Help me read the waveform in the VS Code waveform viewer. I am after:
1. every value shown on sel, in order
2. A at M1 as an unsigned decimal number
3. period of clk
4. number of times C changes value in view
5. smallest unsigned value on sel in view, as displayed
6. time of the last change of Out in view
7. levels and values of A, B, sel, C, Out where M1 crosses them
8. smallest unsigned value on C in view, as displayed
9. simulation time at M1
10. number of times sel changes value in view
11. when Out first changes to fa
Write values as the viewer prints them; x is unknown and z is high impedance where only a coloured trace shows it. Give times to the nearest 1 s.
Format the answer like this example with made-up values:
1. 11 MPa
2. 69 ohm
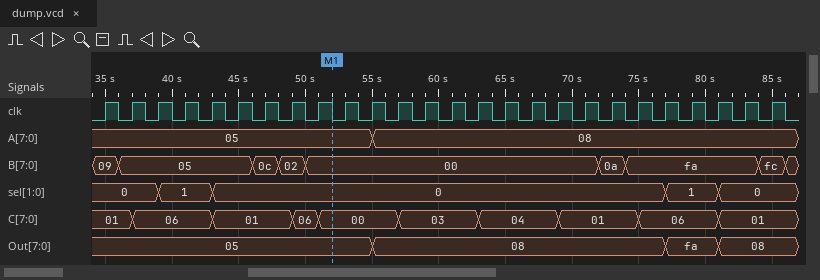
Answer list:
1. 0, 1, 0, 1, 0
2. 5
3. 2 s
4. 9
5. 0
6. 81 s
7. A=05, B=00, sel=0, C=00, Out=05
8. 00
9. 52 s
10. 4
11. 77 s
